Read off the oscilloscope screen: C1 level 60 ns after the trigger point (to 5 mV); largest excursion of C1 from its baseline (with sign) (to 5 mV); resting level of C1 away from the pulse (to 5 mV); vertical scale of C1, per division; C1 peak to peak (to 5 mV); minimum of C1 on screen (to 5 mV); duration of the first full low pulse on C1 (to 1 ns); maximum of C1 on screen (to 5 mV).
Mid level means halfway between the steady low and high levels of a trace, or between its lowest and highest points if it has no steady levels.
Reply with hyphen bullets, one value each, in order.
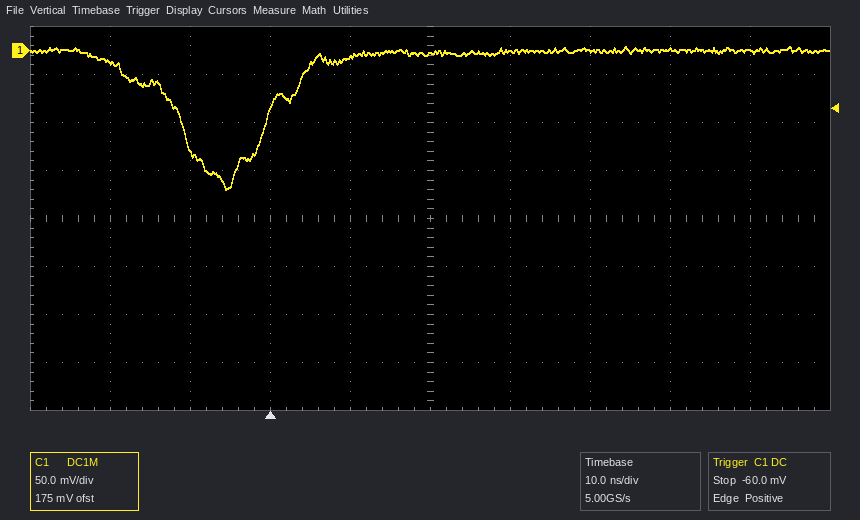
- 0 mV
- -145 mV
- 0 mV
- 50 mV
- 150 mV
- -145 mV
- 11 ns
- 5 mV
